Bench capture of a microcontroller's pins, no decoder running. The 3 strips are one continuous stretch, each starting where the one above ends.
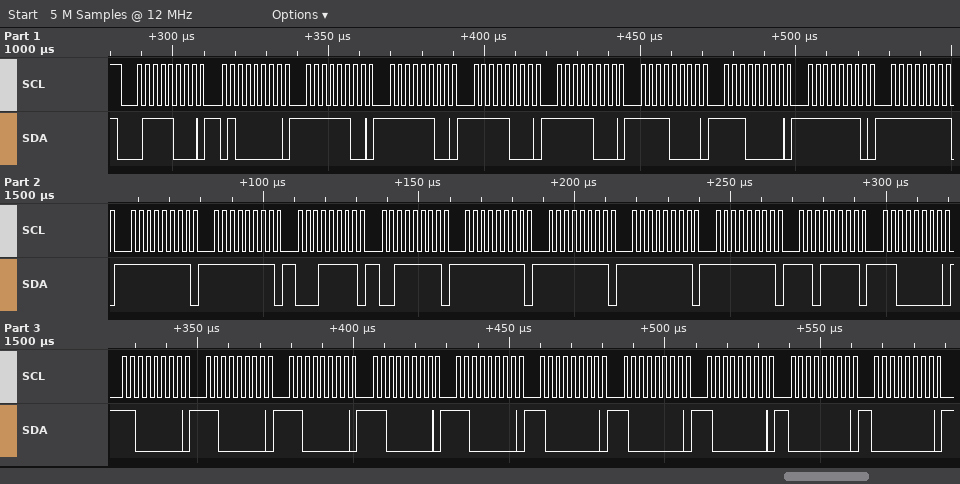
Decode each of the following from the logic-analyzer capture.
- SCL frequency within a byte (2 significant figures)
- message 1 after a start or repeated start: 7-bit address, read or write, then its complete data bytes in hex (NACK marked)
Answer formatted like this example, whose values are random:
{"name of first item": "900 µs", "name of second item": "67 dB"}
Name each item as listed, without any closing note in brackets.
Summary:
{"SCL frequency within a byte": "400 kHz", "message 1 after a start or repeated start: 7-bit address, read or write, then its complete data bytes in hex": "0x3C write: 40 FC FC F8 F8 F0 E0 FE FF FF FF 1F 3F FF FF FF FF DF C0 C0 C0 C0 C0 C0 80 80 80 00 00"}
